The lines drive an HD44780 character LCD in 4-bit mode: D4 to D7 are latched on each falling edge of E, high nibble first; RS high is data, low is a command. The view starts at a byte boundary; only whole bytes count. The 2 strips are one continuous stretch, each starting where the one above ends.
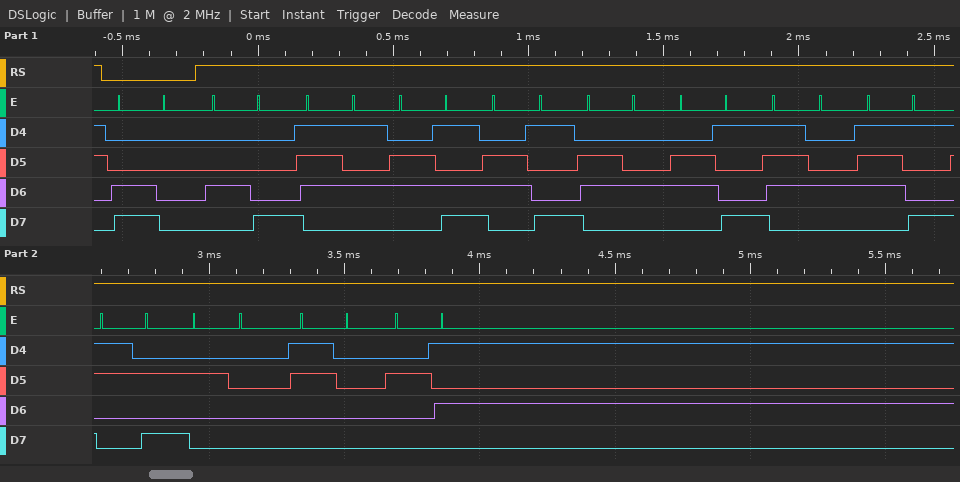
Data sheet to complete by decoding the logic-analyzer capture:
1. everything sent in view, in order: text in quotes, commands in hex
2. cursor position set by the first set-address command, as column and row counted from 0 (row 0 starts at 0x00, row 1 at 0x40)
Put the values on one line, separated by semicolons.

0xC0 "Humidity: 0%"; column 0, row 1
